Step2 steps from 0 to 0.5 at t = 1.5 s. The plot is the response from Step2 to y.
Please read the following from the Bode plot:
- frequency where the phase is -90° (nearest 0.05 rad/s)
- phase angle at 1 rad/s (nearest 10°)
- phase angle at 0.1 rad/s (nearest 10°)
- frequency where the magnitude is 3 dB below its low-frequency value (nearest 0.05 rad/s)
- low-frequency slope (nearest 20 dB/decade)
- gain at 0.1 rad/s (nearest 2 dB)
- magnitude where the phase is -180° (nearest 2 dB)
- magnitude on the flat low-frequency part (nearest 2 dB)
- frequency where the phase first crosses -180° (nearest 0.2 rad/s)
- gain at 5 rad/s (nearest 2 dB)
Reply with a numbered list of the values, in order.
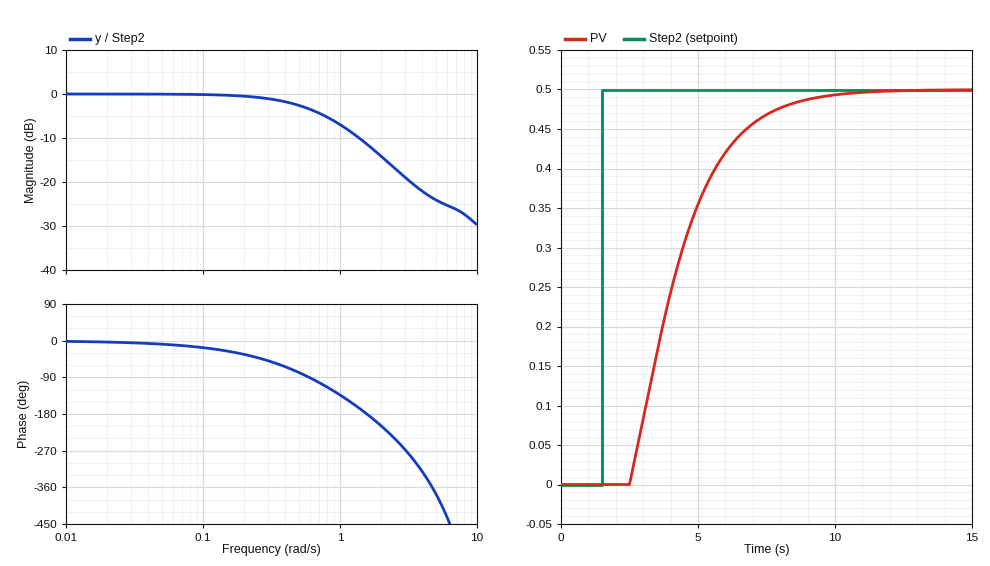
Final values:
1. 0.60 rad/s
2. -130°
3. -20°
4. 0.55 rad/s
5. 0 dB/decade
6. 0 dB
7. -12 dB
8. 0 dB
9. 1.6 rad/s
10. -24 dB
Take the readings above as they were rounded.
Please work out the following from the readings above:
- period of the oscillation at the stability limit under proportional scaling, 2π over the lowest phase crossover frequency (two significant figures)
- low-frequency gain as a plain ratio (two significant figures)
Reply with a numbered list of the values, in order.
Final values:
1. 3.9 s
2. 1.0
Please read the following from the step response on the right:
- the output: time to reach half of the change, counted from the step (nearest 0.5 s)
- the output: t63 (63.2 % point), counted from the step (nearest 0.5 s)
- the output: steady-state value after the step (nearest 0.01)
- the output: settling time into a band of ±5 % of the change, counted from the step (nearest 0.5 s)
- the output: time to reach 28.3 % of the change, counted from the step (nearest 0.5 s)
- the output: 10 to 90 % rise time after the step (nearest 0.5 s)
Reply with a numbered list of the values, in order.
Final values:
1. 2.5 s
2. 3.0 s
3. 0.50
4. 6.5 s
5. 2.0 s
6. 4.0 s
